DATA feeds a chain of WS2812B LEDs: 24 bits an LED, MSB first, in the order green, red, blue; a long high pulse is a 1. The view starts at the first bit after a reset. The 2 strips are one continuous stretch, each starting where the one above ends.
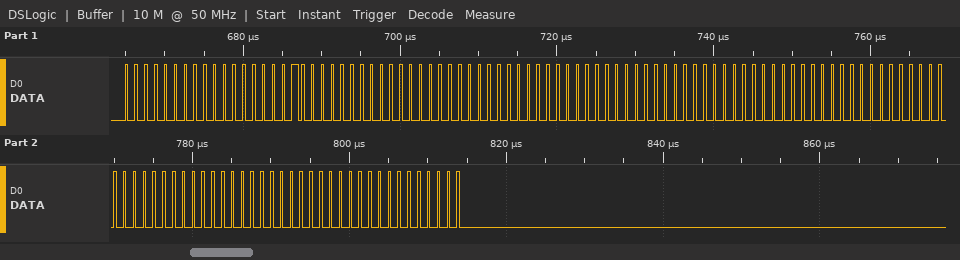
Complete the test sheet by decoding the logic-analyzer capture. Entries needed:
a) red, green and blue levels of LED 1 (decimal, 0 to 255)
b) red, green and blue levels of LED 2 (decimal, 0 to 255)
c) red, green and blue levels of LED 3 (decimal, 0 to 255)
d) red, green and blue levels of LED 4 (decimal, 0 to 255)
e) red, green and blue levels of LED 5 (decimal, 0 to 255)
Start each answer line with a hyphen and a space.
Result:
- 0, 0, 64
- 0, 0, 0
- 0, 0, 0
- 0, 0, 0
- 0, 0, 0
